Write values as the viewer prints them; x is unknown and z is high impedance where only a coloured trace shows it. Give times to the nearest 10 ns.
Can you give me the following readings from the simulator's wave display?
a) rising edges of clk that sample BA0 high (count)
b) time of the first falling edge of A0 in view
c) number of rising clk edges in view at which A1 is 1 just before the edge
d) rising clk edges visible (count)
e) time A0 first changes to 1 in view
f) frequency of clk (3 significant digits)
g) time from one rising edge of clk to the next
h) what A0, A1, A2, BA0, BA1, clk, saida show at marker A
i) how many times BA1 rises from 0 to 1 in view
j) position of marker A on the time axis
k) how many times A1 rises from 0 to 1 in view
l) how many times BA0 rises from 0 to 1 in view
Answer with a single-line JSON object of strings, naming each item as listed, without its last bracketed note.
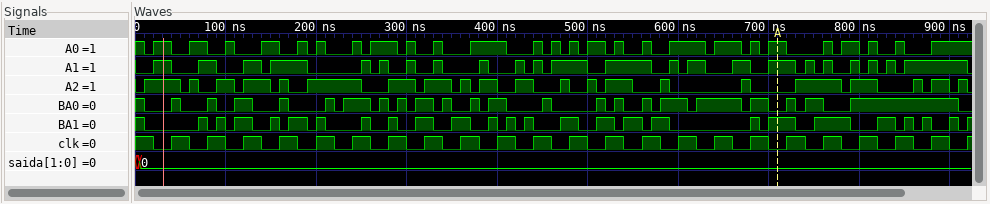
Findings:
{"rising edges of clk that sample BA0 high": "12", "time of the first falling edge of A0 in view": "10 ns", "number of rising clk edges in view at which A1 is 1 just before the edge": "13", "rising clk edges visible": "23", "time A0 first changes to 1 in view": "20 ns", "frequency of clk": "25.0 MHz", "time from one rising edge of clk to the next": "40 ns", "what A0, A1, A2, BA0, BA1, clk, saida show at marker A": "A0=1, A1=1, A2=0, BA0=0, BA1=1, clk=0, saida=0", "how many times BA1 rises from 0 to 1 in view": "25", "position of marker A on the time axis": "710 ns", "how many times A1 rises from 0 to 1 in view": "23", "how many times BA0 rises from 0 to 1 in view": "22"}
